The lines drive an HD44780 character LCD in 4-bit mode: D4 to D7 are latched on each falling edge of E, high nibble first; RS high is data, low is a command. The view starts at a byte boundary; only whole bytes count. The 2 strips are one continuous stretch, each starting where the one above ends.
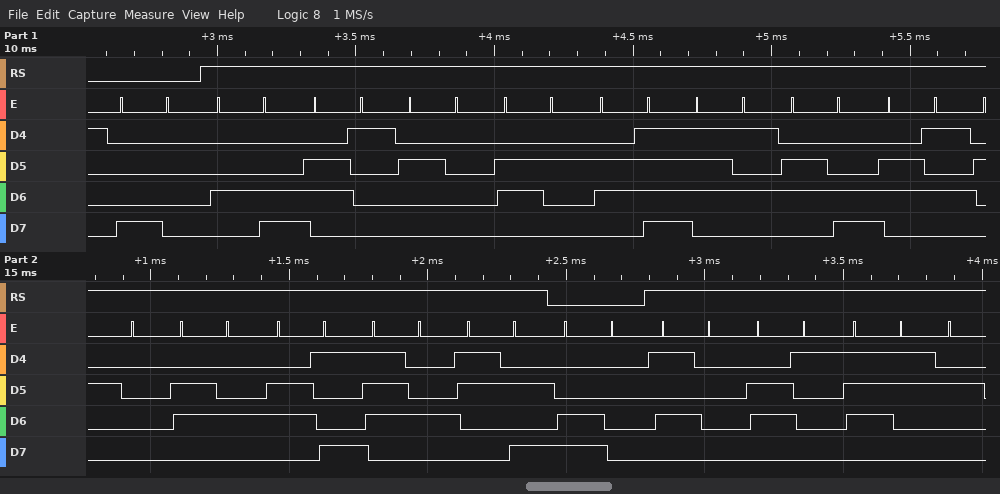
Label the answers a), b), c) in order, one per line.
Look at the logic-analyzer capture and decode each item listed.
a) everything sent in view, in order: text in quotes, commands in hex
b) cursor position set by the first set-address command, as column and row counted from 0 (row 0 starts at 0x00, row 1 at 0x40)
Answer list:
a) 0x80 "La boule dit:" 0xC0 "Pas"
b) column 0, row 0
